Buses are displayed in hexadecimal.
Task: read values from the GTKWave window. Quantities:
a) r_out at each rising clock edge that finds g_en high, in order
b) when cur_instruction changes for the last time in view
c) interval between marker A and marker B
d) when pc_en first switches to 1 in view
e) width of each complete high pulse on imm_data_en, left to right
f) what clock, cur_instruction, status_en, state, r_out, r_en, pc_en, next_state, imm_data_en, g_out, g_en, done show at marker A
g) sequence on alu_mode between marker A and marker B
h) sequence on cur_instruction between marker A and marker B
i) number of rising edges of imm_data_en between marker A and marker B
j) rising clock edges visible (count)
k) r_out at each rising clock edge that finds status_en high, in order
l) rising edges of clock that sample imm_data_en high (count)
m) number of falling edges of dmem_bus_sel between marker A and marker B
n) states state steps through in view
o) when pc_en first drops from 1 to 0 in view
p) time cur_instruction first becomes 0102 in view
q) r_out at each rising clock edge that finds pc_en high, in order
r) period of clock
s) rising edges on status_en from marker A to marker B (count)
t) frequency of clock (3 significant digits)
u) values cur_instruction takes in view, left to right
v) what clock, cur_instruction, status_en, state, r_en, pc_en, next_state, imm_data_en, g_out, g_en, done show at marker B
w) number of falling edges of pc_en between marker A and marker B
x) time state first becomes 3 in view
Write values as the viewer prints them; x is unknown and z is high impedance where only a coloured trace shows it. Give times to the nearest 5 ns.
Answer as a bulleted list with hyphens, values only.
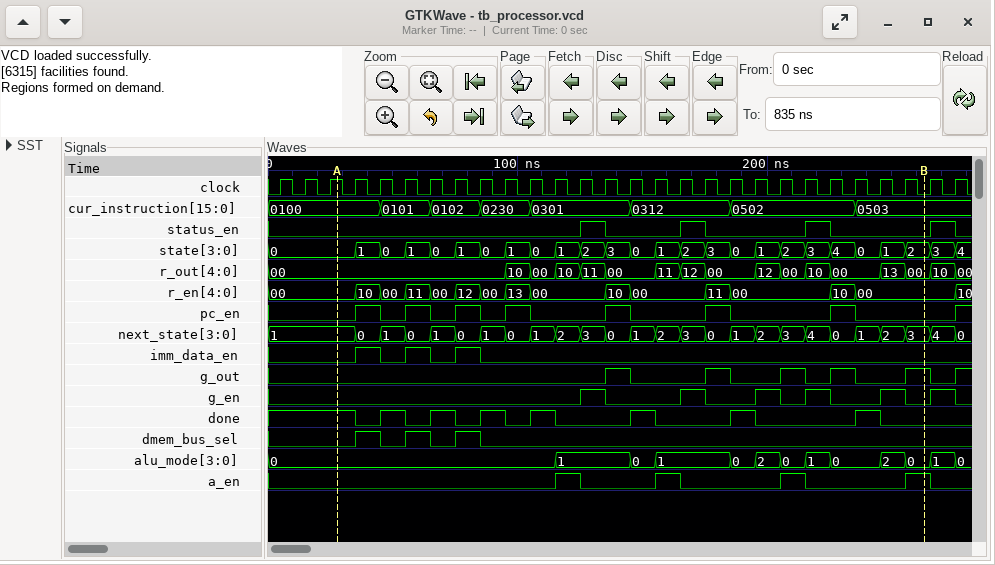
- 11, 12, 12, 10, 13, 10
- 235 ns
- 235 ns
- 35 ns
- 10 ns, 10 ns, 10 ns
- clock=1, cur_instruction=0100, status_en=0, state=0, r_out=00, r_en=00, pc_en=0, next_state=1, imm_data_en=0, g_out=0, g_en=0, done=1
- 0, 1, 0, 1, 0, 2, 0, 1, 0, 2, 0
- 0100, 0101, 0102, 0230, 0301, 0312, 0502, 0503
- 3
- 28
- 11, 12, 10, 10
- 3
- 3
- 0, 1, 0, 1, 0, 1, 0, 1, 0, 1, 2, 3, 0, 1, 2, 3, 0, 1, 2, 3, 4, 0, 1, 2, 3, 4
- 45 ns
- 65 ns
- 00, 00, 00, 10, 00, 00, 00
- 10 ns
- 3
- 100 MHz
- 0100, 0101, 0102, 0230, 0301, 0312, 0502, 0503
- clock=0, cur_instruction=0503, status_en=0, state=2, r_en=00, pc_en=0, next_state=3, imm_data_en=0, g_out=1, g_en=0, done=0
- 7
- 135 ns
